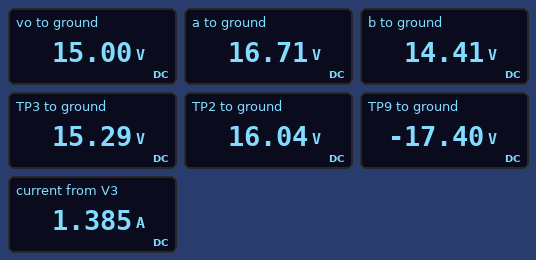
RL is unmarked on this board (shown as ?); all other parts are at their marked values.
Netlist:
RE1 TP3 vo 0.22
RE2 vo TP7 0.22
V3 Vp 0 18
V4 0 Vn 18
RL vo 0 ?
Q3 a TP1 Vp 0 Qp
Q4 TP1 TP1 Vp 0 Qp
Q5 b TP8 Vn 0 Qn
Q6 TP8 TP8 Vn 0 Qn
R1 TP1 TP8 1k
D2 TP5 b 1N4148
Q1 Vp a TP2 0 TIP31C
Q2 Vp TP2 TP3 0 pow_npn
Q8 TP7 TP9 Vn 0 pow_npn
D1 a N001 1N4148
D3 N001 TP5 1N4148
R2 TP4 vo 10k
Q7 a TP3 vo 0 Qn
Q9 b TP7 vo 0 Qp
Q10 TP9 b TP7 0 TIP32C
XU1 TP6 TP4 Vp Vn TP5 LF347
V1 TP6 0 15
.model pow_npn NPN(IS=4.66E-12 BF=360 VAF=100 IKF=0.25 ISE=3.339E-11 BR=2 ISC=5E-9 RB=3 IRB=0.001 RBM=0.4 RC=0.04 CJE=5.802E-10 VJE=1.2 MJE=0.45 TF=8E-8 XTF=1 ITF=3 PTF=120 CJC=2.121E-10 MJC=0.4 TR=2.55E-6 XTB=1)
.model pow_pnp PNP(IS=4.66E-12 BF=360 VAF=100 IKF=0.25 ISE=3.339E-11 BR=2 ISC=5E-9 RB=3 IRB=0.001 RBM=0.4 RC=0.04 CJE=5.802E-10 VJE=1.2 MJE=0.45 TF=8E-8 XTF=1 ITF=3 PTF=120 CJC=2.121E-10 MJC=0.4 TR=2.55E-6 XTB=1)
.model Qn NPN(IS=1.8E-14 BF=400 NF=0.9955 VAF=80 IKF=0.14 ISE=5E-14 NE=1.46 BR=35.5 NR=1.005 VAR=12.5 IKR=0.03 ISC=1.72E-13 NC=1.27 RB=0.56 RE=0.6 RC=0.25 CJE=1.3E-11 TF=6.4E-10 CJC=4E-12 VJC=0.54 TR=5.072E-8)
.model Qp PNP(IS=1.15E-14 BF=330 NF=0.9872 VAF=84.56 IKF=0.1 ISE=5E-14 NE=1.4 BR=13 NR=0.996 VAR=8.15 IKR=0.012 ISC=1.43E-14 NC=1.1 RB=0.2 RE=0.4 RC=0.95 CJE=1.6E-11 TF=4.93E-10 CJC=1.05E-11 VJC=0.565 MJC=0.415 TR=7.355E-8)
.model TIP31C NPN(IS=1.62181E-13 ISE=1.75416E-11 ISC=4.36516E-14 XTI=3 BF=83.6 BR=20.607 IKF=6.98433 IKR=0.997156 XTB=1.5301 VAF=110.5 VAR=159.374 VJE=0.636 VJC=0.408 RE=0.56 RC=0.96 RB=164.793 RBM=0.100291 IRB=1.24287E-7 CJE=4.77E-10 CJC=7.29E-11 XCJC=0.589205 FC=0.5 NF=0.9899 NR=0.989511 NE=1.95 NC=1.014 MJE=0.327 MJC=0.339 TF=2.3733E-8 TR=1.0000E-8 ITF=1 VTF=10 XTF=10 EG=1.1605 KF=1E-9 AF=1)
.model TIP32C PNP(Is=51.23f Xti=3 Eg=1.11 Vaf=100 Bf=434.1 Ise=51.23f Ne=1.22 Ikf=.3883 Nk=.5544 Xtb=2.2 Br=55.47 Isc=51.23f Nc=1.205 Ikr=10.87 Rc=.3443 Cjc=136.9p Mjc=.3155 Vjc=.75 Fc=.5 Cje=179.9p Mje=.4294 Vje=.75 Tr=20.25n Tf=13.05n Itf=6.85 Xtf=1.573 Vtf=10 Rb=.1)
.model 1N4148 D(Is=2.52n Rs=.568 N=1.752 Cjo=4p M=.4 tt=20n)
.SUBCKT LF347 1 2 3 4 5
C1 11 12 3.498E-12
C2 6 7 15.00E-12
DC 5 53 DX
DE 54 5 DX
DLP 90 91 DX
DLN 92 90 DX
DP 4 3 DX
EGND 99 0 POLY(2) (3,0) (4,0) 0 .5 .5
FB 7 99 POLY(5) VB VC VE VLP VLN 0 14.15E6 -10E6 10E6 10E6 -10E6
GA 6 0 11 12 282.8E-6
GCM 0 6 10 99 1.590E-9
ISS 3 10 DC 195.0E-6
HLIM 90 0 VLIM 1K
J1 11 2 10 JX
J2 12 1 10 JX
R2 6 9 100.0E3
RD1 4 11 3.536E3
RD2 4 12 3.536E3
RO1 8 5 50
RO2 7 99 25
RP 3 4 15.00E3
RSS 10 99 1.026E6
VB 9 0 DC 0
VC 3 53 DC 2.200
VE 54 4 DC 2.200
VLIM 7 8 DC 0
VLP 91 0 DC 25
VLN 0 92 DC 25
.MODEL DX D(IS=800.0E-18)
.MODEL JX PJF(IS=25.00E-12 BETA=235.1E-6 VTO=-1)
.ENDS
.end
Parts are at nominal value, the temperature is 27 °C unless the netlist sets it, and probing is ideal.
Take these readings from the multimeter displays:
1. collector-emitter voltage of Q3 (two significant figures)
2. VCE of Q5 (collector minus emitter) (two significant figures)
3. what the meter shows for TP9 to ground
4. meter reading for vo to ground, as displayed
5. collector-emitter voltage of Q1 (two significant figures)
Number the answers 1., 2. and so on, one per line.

1. -1.3 V
2. 32 V
3. -17.40 V
4. 15.00 V
5. 2.0 V
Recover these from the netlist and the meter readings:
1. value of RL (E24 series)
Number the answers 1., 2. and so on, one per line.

1. 12 Ω
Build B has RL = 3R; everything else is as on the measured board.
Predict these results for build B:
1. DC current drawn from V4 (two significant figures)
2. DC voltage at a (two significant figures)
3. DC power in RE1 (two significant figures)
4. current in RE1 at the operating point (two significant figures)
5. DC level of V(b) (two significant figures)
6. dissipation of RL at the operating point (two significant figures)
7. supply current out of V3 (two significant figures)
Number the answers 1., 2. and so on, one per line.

1. 78 mA
2. 12 V
3. 2.4 W
4. 3.3 A
5. 10 V
6. 33 W
7. 3.4 A
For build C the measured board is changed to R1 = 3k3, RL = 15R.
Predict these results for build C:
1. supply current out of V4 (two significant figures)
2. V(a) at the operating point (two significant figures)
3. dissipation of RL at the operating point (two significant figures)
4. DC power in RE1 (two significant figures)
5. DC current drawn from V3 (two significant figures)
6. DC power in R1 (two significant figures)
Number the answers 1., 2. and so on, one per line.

1. 28 mA
2. 17 V
3. 15 W
4. 220 mW
5. 1.0 A
6. 360 mW
